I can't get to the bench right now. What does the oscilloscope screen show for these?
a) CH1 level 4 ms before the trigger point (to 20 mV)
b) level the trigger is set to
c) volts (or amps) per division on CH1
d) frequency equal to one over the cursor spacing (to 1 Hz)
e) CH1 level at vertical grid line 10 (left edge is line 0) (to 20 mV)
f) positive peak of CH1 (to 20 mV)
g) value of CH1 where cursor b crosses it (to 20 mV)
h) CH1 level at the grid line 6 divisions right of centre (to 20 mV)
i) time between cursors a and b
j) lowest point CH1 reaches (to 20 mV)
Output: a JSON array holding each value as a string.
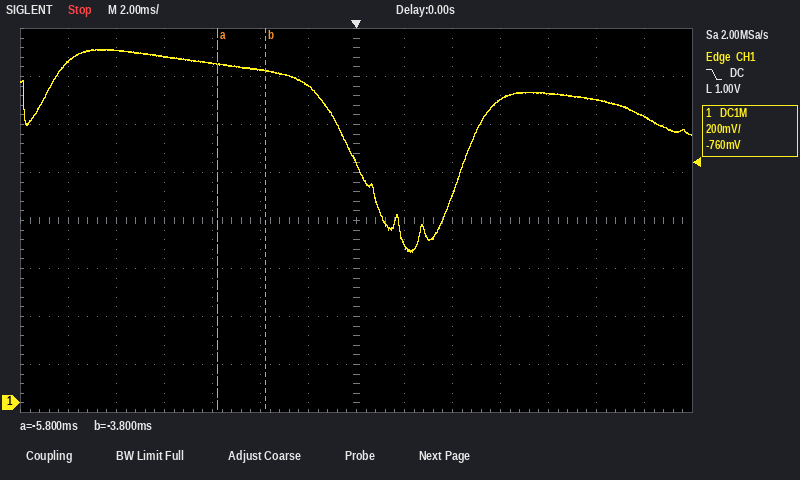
["1.38 V", "1.00 V", "200 mV", "500 Hz", "1.26 V", "1.48 V", "1.38 V", "1.20 V", "2.0 ms", "620 mV"]
